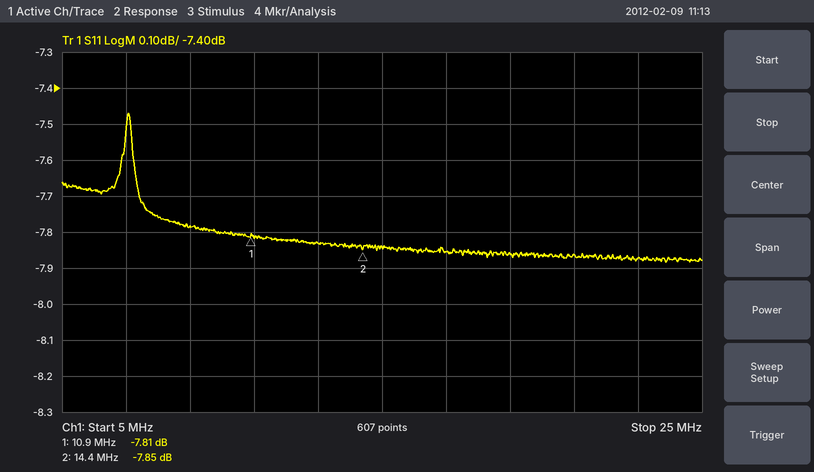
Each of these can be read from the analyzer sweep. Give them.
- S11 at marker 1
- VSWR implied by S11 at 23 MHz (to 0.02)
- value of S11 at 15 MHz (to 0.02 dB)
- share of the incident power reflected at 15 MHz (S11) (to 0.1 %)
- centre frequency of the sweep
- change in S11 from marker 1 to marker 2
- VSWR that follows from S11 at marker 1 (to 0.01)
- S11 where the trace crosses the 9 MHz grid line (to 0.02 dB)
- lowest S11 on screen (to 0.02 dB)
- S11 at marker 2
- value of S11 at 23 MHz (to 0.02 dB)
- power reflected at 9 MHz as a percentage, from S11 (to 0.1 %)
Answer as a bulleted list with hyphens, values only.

- -7.81 dB
- 2.36
- -7.84 dB
- 16.4 %
- 15 MHz
- -0.04 dB
- 2.37
- -7.78 dB
- -7.88 dB
- -7.85 dB
- -7.88 dB
- 16.7 %
